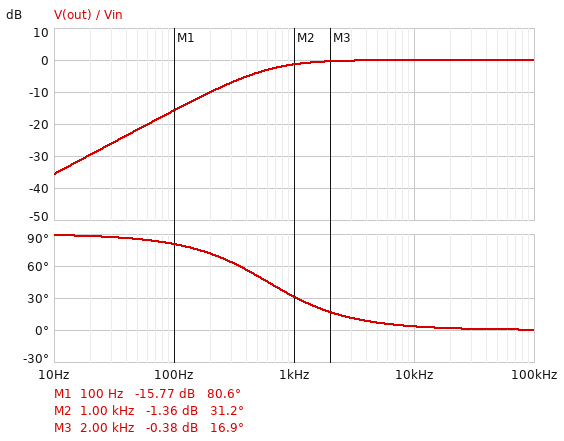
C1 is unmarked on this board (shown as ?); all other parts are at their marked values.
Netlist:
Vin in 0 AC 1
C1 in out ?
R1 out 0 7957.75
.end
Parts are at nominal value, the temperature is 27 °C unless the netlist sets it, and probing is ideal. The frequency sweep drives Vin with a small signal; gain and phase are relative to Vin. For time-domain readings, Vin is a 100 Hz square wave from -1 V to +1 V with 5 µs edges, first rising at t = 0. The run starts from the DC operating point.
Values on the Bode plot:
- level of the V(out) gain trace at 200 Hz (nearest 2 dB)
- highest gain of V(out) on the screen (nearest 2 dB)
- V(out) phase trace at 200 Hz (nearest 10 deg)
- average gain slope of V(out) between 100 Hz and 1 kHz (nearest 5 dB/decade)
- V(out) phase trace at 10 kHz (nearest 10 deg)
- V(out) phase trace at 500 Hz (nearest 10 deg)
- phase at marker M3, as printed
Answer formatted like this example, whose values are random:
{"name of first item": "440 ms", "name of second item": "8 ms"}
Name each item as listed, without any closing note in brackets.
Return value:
{"level of the V(out) gain trace at 200 Hz": "-10 dB", "highest gain of V(out) on the screen": "0 dB", "V(out) phase trace at 200 Hz": "70 deg", "average gain slope of V(out) between 100 Hz and 1 kHz": "15 dB/decade", "V(out) phase trace at 10 kHz": "0 deg", "V(out) phase trace at 500 Hz": "50 deg", "phase at marker M3, as printed": "16.9 deg"}
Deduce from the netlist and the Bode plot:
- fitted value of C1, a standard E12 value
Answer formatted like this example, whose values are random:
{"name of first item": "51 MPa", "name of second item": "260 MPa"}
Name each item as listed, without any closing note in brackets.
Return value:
{"fitted value of C1, a standard E12 value": "33 nF"}
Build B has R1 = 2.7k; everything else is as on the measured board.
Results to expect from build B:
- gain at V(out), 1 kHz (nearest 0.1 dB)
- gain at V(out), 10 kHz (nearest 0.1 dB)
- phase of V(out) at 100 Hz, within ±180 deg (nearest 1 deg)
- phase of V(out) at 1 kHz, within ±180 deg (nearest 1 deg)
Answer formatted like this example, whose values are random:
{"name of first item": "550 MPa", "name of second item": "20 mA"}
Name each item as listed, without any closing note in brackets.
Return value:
{"gain at V(out), 1 kHz": "-6.2 dB", "gain at V(out), 10 kHz": "-0.1 dB", "phase of V(out) at 100 Hz, within ±180 deg": "87 deg", "phase of V(out) at 1 kHz, within ±180 deg": "61 deg"}
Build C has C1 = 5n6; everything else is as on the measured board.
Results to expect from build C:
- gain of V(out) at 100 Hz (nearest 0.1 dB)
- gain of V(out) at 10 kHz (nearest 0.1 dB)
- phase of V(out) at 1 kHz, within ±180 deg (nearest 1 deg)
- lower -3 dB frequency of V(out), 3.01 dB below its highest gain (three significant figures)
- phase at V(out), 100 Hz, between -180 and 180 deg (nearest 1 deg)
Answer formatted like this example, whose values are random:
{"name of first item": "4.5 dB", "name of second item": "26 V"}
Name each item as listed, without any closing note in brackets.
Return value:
{"gain of V(out) at 100 Hz": "-31.1 dB", "gain of V(out) at 10 kHz": "-0.5 dB", "phase of V(out) at 1 kHz, within ±180 deg": "74 deg", "lower -3 dB frequency of V(out), 3.01 dB below its highest gain": "3.57 kHz", "phase at V(out), 100 Hz, between -180 and 180 deg": "88 deg"}
